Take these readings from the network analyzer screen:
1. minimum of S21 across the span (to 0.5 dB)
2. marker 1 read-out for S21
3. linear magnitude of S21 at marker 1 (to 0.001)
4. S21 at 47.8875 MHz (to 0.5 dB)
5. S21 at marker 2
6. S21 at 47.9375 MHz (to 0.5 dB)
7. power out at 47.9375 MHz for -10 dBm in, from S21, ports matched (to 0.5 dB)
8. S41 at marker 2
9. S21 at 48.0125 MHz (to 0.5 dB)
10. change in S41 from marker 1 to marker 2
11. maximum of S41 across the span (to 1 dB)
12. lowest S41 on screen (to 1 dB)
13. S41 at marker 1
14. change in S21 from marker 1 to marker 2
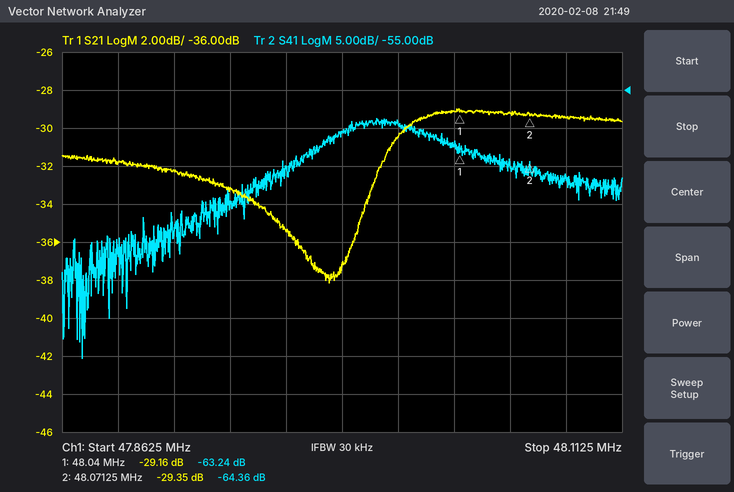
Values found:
-38.0 dB
-29.16 dB
0.035
-32.0 dB
-29.35 dB
-33.0 dB
-43.0 dBm
-64.36 dB
-30.5 dB
-1.12 dB
-59 dB
-90 dB
-63.24 dB
-0.19 dB
